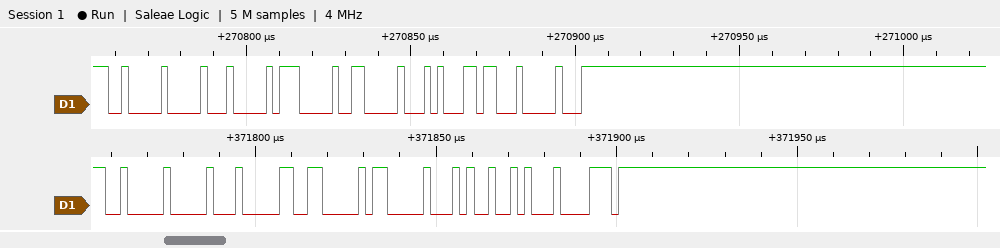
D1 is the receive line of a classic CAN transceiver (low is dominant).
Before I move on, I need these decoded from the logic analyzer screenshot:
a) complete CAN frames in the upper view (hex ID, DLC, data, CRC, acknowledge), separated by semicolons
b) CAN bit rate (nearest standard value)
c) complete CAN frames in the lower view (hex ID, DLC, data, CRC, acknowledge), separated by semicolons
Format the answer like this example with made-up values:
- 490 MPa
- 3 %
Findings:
- ID 200, DLC 4, data 0E 03 00 A3, CRC 3100, NACK
- 500 kbit/s
- ID 200, DLC 4, data 13 03 00 A4, CRC 510E, NACK
